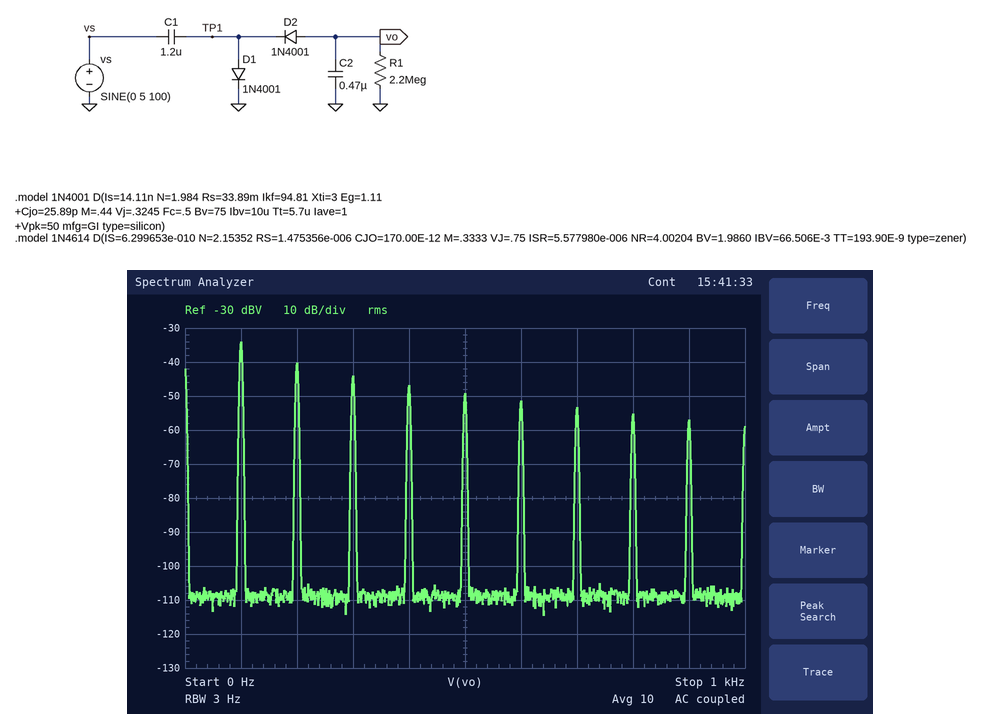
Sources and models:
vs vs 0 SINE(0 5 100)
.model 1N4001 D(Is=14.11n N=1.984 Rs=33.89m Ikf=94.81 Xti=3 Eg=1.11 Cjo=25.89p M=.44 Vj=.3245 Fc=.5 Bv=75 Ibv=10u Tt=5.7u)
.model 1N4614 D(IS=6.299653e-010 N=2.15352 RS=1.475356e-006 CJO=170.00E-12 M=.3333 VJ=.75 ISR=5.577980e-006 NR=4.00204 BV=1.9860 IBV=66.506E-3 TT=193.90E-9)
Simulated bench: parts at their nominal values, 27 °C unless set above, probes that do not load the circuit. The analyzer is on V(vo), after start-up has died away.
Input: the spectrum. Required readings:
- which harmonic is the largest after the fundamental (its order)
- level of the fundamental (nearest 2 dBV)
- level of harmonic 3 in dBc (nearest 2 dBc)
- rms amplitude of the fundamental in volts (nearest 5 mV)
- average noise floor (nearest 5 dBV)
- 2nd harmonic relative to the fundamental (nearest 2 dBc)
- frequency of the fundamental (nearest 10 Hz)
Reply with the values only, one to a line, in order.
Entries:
2
-34 dBV
-10 dBc
20 mV
-110 dBV
-6 dBc
100 Hz
